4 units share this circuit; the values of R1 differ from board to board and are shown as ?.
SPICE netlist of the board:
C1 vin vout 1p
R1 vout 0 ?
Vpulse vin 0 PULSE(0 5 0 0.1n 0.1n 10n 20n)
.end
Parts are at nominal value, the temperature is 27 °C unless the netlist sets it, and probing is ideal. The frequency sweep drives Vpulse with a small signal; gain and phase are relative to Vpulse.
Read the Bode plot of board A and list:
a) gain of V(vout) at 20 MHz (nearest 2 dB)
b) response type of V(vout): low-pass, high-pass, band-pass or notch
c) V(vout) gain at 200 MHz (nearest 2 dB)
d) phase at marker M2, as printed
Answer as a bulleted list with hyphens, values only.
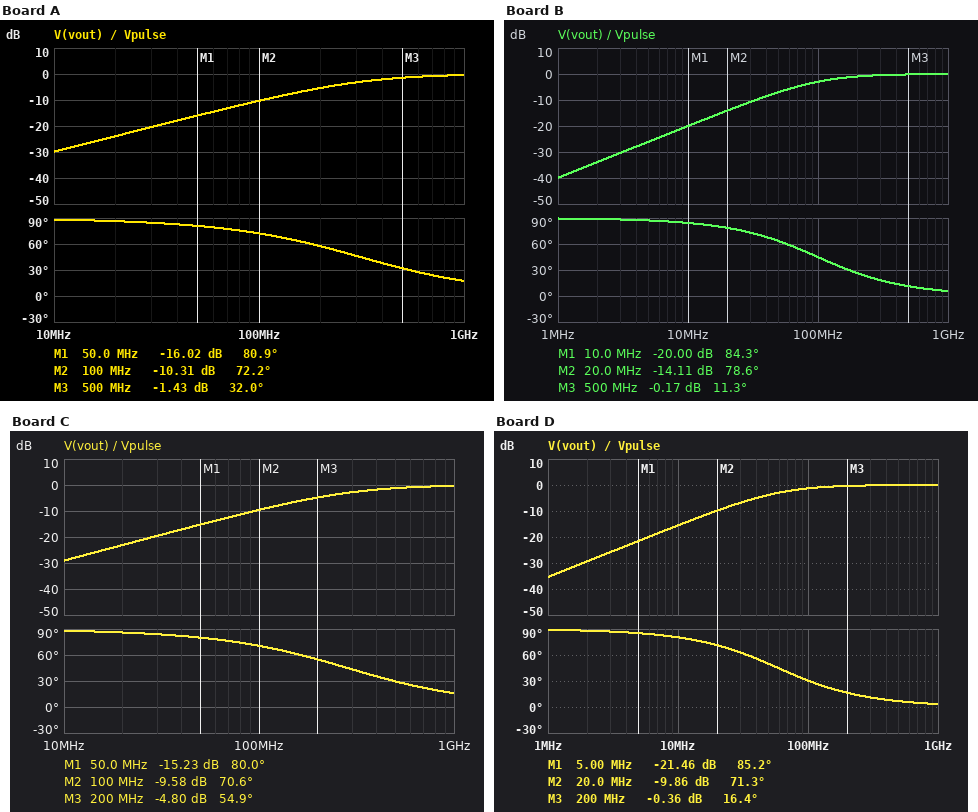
- -24 dB
- high-pass
- -6 dB
- 72.2 deg
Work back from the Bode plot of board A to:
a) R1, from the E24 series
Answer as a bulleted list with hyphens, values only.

- 510 Ω
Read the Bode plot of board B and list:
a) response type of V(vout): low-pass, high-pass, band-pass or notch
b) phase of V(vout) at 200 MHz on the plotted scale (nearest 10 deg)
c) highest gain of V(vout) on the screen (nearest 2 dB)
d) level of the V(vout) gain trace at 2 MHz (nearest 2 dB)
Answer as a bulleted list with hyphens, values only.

- high-pass
- 30 deg
- 0 dB
- -34 dB
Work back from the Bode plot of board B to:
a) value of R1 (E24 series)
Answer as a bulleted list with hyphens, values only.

- 1.6 kΩ
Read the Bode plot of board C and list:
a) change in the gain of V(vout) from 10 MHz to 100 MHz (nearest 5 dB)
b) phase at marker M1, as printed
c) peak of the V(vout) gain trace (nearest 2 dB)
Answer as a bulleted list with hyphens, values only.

- 20 dB
- 80.0 deg
- 0 dB
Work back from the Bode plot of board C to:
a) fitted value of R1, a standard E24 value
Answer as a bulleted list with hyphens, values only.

- 560 Ω
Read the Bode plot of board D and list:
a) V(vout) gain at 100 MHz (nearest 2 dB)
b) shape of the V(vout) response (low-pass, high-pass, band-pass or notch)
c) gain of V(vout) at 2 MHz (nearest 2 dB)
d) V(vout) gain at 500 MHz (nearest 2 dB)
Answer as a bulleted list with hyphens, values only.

- -2 dB
- high-pass
- -30 dB
- 0 dB
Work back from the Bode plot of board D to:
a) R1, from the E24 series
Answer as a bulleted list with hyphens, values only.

- 2.7 kΩ
